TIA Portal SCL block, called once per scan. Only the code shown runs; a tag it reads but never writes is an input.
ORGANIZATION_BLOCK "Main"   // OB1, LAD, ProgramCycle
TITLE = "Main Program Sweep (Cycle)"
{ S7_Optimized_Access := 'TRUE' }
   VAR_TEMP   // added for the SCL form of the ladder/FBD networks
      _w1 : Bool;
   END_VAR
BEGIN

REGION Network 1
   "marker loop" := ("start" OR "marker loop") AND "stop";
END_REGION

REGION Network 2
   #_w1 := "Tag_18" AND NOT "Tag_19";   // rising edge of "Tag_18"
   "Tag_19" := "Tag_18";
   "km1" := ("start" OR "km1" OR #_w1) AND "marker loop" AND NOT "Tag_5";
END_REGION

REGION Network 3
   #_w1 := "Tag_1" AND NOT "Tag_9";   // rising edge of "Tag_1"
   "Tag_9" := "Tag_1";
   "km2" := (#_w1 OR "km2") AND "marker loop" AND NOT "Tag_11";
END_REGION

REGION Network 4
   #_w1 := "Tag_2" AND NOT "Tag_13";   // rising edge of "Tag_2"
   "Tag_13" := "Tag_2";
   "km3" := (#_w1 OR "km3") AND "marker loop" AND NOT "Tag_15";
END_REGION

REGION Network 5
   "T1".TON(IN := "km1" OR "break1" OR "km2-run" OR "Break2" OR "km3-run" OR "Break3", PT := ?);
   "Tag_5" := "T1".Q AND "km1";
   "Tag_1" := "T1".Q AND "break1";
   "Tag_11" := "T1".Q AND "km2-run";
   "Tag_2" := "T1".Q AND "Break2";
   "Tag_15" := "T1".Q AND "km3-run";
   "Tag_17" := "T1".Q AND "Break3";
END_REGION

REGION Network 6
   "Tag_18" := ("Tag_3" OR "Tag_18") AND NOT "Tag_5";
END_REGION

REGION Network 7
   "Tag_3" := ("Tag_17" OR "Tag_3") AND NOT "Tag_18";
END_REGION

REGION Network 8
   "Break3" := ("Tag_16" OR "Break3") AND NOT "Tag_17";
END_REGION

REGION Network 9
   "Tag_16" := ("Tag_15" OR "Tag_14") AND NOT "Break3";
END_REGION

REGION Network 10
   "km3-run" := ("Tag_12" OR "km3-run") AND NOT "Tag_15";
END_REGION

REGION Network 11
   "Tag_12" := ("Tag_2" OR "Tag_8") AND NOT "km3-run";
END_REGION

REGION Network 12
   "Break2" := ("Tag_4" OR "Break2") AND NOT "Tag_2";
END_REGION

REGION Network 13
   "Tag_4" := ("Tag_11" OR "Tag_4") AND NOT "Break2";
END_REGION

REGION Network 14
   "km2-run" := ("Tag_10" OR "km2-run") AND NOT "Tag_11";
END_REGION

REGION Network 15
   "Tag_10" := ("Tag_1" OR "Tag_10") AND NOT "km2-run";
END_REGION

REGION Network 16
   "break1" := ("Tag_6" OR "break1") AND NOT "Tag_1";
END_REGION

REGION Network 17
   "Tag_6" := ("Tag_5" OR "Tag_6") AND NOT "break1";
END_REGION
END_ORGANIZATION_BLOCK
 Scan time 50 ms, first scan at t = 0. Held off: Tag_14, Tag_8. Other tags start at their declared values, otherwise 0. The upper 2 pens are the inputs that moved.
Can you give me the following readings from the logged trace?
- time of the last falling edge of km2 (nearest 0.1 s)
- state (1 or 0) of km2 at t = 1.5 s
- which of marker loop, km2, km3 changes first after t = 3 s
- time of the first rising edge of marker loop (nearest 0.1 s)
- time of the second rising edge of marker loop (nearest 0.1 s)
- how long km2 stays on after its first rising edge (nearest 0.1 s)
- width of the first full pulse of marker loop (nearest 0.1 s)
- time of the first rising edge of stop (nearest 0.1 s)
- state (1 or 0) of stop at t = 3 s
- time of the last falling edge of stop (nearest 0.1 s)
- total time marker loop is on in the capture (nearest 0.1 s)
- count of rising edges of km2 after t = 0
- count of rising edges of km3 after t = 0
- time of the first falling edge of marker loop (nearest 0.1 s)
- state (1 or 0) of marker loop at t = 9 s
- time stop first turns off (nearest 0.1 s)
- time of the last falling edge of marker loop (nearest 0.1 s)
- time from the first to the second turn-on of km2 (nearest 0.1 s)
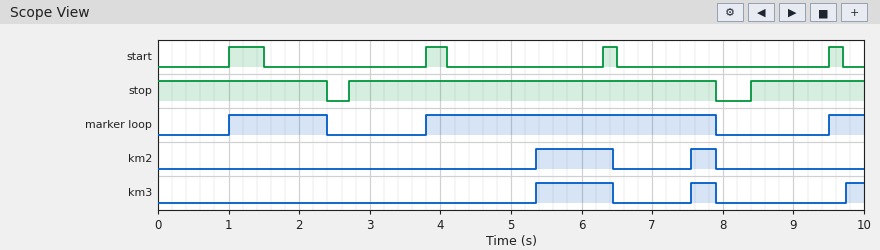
7.9 s
0
marker loop
1.0 s
3.8 s
1.1 s
1.4 s
2.7 s
1
7.9 s
6.0 s
2
3
2.4 s
0
2.4 s
7.9 s
2.2 s
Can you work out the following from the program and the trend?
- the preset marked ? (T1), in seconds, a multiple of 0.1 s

1.0 s
